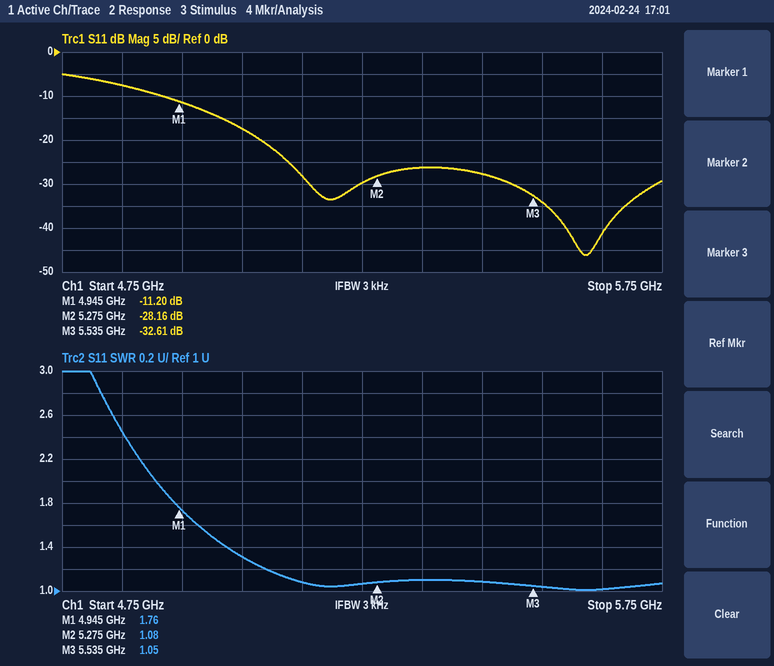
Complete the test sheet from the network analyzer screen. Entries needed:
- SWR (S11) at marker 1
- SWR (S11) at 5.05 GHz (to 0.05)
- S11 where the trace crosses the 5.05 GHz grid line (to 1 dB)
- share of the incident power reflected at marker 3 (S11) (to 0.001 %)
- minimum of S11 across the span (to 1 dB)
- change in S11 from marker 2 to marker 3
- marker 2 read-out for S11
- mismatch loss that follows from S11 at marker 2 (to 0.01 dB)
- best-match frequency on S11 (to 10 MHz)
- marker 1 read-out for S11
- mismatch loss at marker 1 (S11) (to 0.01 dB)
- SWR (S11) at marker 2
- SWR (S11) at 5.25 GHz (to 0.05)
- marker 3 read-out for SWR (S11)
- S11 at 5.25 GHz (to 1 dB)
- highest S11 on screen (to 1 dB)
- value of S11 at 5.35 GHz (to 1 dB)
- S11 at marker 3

1.76
1.30
-17 dB
0.055 %
-46 dB
-4.45 dB
-28.16 dB
0.01 dB
5.62 GHz
-11.20 dB
0.34 dB
1.08
1.05
1.05
-30 dB
-5 dB
-26 dB
-32.61 dB
